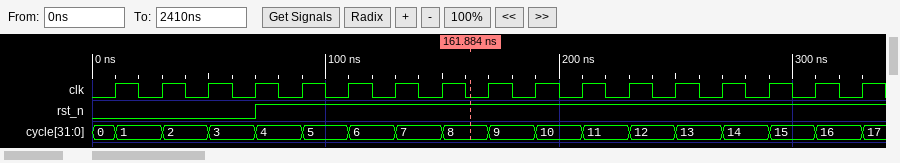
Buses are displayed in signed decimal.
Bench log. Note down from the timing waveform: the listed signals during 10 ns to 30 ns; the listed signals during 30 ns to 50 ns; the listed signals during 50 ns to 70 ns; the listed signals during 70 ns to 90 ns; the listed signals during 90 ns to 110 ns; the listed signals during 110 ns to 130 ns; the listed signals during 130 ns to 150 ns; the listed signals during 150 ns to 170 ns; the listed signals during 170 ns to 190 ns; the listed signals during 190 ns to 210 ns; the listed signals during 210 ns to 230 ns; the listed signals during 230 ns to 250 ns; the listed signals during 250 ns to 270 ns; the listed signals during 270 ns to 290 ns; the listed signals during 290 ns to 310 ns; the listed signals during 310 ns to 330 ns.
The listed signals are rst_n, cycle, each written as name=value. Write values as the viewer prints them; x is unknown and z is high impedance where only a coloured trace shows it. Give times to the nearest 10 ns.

rst_n=0, cycle=1
rst_n=0, cycle=2
rst_n=0, cycle=3
rst_n=1, cycle=4
rst_n=1, cycle=5
rst_n=1, cycle=6
rst_n=1, cycle=7
rst_n=1, cycle=8
rst_n=1, cycle=9
rst_n=1, cycle=10
rst_n=1, cycle=11
rst_n=1, cycle=12
rst_n=1, cycle=13
rst_n=1, cycle=14
rst_n=1, cycle=15
rst_n=1, cycle=16
